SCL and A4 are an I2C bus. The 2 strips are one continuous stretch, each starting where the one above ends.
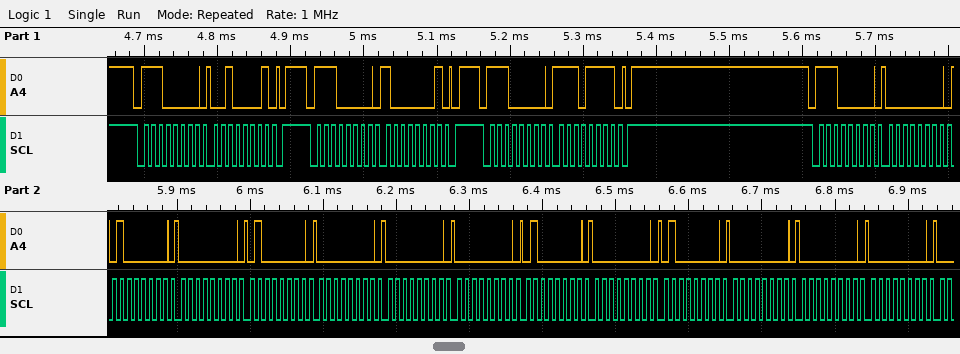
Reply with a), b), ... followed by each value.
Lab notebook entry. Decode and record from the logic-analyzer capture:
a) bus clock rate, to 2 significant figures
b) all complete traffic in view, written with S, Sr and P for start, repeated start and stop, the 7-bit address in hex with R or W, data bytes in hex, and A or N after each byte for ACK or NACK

a) 100 kHz
b) S 70W A 21 A P S 70W A 81 A P S 70W A EF A P S 70W A 00 A 40 A 00 A 40 A 00 A 00 A 00 A 40 A 00 A 40 A 00 A 00 A 00 A
